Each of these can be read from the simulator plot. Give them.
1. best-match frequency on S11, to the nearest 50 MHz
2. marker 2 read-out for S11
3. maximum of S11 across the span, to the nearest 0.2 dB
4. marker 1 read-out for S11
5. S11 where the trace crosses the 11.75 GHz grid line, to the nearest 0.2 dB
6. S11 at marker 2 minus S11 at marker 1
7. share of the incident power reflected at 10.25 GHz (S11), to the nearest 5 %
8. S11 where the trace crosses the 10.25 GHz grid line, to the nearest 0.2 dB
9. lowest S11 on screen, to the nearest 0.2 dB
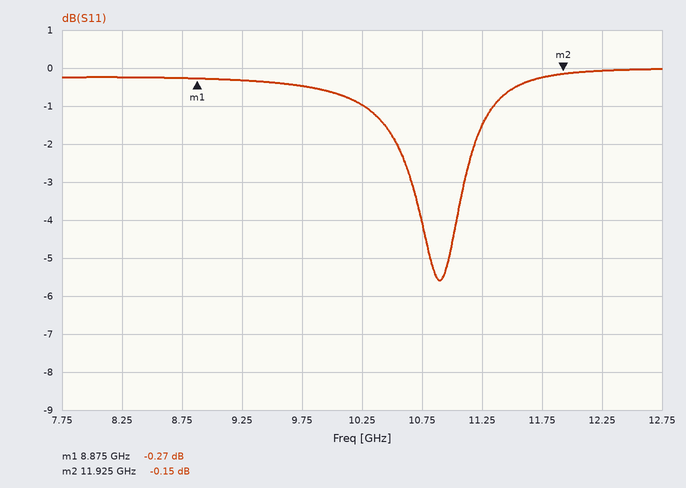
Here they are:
10.90 GHz
-0.15 dB
0.0 dB
-0.27 dB
-0.2 dB
0.12 dB
80 %
-1.0 dB
-5.6 dB
